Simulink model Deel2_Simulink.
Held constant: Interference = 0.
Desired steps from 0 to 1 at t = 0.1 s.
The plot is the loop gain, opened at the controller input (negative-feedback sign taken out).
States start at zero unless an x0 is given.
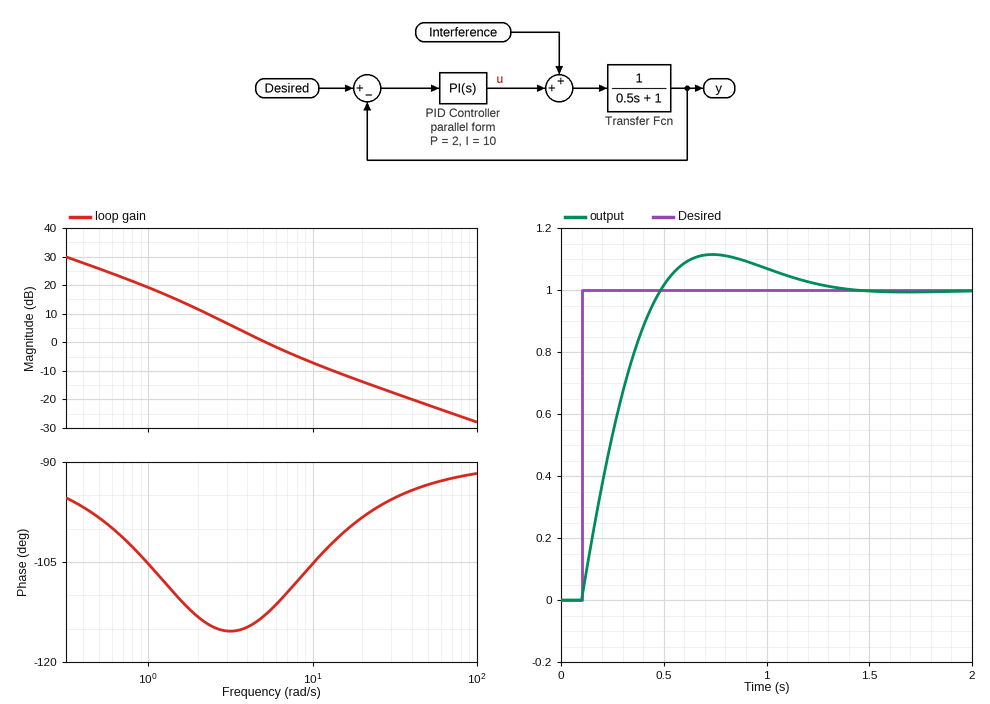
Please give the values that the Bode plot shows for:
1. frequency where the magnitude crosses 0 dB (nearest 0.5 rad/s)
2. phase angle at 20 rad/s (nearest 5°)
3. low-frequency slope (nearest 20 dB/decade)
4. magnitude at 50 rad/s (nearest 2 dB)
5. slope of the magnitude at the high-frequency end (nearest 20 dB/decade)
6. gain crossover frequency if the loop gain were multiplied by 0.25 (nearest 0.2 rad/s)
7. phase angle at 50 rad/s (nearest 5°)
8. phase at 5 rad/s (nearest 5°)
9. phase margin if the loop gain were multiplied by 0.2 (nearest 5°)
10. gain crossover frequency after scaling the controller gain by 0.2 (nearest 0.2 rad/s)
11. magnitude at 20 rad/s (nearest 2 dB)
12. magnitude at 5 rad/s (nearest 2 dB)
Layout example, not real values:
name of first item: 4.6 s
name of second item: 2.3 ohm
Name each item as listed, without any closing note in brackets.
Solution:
frequency where the magnitude crosses 0 dB: 5.0 rad/s
phase angle at 20 rad/s: -100°
low-frequency slope: -20 dB/decade
magnitude at 50 rad/s: -22 dB
slope of the magnitude at the high-frequency end: -20 dB/decade
gain crossover frequency if the loop gain were multiplied by 0.25: 2.0 rad/s
phase angle at 50 rad/s: -95°
phase at 5 rad/s: -115°
phase margin if the loop gain were multiplied by 0.2: 70°
gain crossover frequency after scaling the controller gain by 0.2: 1.6 rad/s
magnitude at 20 rad/s: -14 dB
magnitude at 5 rad/s: 0 dB
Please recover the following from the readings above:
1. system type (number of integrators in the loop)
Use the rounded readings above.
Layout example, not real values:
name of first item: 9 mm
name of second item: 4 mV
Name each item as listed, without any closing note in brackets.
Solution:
system type: 1
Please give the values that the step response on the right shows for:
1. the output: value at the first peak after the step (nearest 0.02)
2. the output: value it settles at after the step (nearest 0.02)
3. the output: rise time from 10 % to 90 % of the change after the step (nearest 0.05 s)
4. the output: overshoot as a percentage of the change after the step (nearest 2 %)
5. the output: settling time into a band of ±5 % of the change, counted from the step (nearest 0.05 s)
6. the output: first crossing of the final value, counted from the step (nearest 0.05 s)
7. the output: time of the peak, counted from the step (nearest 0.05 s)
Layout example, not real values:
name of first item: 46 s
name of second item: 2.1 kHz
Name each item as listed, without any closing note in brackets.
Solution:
the output: value at the first peak after the step: 1.12
the output: value it settles at after the step: 1.00
the output: rise time from 10 % to 90 % of the change after the step: 0.30 s
the output: overshoot as a percentage of the change after the step: 12 %
the output: settling time into a band of ±5 % of the change, counted from the step: 1.00 s
the output: first crossing of the final value, counted from the step: 0.40 s
the output: time of the peak, counted from the step: 0.65 s
